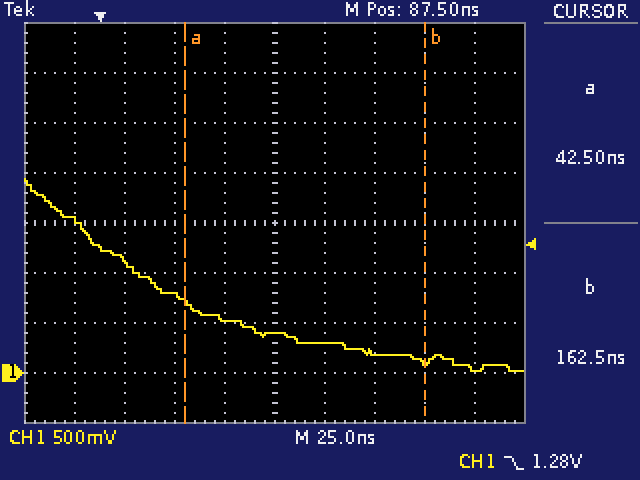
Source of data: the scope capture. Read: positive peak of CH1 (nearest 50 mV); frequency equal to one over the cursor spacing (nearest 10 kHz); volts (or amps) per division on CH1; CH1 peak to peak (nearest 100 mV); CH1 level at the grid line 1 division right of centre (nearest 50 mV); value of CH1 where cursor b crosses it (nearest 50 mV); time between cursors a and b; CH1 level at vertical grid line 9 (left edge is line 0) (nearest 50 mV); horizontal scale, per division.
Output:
1.95 V
8.33 MHz
500 mV
1.90 V
300 mV
100 mV
120.0 ns
50 mV
25 ns
